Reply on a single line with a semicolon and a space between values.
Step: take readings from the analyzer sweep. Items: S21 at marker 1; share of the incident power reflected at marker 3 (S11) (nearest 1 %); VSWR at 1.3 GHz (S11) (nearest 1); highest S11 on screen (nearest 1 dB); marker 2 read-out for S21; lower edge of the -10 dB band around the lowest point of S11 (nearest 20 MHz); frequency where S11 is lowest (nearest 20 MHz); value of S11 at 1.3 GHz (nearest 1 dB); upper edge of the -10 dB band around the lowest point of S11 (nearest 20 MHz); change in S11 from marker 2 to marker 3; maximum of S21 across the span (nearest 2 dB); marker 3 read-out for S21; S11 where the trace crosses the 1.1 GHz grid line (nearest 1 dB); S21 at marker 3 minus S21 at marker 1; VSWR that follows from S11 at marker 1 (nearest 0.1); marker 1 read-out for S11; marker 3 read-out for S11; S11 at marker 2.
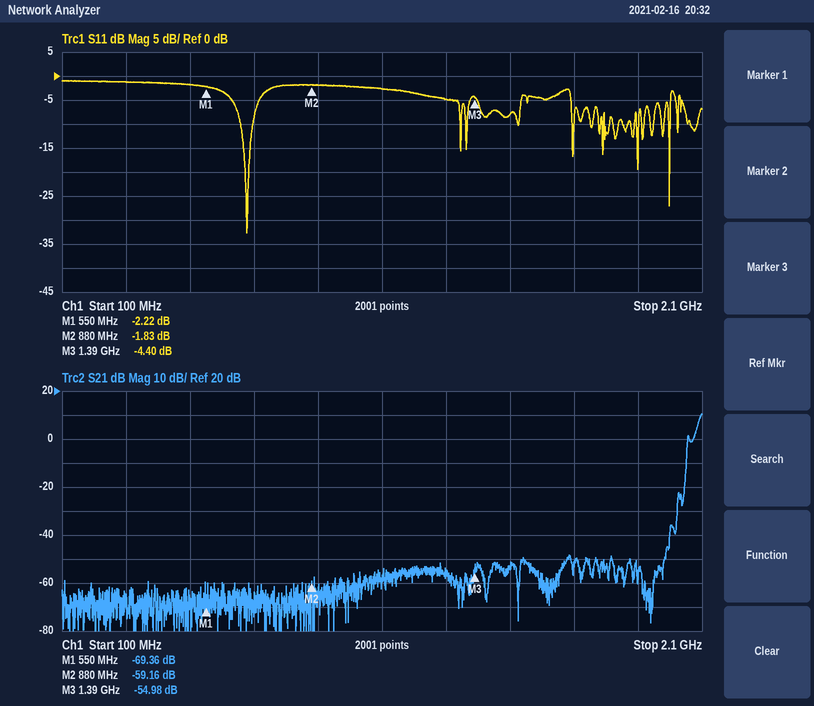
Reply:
-69.36 dB; 36 %; 4; -1 dB; -59.16 dB; 660 MHz; 680 MHz; -5 dB; 700 MHz; -2.57 dB; 10 dB; -54.98 dB; -3 dB; 14.38 dB; 7.9; -2.22 dB; -4.40 dB; -1.83 dB
